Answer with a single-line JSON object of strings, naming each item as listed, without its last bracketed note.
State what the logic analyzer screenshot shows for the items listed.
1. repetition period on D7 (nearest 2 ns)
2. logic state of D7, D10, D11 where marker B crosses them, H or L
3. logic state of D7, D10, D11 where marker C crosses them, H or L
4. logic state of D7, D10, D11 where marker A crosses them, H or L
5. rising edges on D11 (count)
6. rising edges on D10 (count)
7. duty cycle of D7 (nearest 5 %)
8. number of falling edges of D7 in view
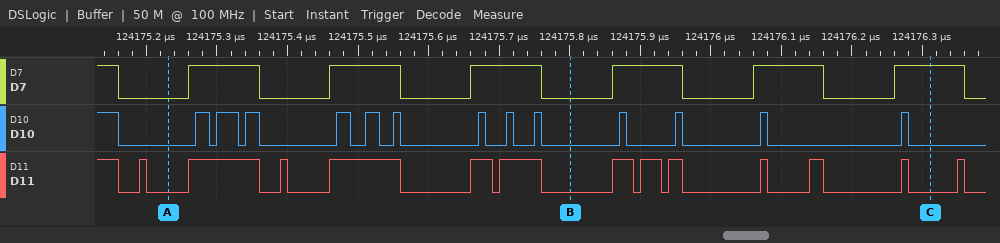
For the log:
{"repetition period on D7": "200 ns", "logic state of D7, D10, D11 where marker B crosses them, H or L": "D7=L, D10=L, D11=L", "logic state of D7, D10, D11 where marker C crosses them, H or L": "D7=H, D10=L, D11=L", "logic state of D7, D10, D11 where marker A crosses them, H or L": "D7=L, D10=L, D11=L", "rising edges on D11": "13", "rising edges on D10": "13", "duty cycle of D7": "50 %", "number of falling edges of D7 in view": "7"}
